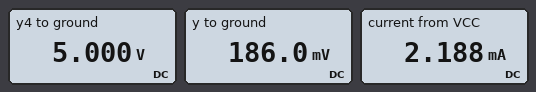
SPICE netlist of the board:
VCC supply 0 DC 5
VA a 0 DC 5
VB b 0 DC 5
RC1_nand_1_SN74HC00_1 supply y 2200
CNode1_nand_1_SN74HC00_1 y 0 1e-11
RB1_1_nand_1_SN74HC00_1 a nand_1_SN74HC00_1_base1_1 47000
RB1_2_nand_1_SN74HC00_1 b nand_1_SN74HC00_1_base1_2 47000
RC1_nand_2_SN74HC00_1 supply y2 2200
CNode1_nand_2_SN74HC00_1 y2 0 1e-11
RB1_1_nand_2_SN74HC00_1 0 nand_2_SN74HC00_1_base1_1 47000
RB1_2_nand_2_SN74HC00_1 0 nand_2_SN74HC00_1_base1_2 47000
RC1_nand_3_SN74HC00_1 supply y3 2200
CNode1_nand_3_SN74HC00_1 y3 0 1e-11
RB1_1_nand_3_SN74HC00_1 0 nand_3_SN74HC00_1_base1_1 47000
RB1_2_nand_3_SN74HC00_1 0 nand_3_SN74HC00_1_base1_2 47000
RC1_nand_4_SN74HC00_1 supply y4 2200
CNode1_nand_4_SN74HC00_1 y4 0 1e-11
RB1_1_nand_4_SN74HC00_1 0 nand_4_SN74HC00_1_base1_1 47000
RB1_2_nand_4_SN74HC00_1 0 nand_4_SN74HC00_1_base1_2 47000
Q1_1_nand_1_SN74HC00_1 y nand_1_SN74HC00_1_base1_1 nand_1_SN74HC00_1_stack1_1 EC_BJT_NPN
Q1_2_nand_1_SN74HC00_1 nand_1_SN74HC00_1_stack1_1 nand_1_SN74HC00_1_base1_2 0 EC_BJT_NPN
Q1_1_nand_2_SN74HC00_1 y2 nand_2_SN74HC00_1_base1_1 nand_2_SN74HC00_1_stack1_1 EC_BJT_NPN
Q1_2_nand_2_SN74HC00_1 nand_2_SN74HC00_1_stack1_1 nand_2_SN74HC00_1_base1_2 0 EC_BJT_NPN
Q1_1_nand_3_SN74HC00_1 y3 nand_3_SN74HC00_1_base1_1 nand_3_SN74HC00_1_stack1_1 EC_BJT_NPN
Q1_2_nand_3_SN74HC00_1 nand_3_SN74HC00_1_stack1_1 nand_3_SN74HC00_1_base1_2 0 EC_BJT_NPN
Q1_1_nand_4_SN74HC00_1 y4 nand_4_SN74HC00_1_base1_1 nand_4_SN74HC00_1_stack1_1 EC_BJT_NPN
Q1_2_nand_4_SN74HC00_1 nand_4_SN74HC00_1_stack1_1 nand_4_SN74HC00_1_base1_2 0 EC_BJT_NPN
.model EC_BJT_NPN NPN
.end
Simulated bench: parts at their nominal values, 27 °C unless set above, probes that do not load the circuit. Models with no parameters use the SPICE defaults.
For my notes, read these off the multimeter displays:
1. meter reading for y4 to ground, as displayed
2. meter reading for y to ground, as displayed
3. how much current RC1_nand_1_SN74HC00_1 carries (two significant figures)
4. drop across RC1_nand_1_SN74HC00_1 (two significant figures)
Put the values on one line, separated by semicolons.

5.000 V; 186.0 mV; 2.2 mA; 4.8 V
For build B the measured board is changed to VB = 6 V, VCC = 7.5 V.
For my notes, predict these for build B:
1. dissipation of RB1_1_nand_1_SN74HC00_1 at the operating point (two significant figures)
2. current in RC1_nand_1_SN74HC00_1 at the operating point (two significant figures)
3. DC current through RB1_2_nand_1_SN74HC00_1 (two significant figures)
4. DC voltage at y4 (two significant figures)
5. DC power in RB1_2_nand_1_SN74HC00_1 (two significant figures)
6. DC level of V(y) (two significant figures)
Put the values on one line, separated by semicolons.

360 µW; 3.3 mA; 110 µA; 7.5 V; 570 µW; 210 mV
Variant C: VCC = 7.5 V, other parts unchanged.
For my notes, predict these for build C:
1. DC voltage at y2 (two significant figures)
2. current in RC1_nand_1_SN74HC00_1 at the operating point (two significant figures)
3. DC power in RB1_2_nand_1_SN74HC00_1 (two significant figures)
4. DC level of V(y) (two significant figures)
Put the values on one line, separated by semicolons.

7.5 V; 3.3 mA; 370 µW; 220 mV
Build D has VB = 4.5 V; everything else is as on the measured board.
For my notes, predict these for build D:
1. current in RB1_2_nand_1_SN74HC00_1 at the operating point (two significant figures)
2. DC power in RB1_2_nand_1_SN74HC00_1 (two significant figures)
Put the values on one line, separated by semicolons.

79 µA; 290 µW
